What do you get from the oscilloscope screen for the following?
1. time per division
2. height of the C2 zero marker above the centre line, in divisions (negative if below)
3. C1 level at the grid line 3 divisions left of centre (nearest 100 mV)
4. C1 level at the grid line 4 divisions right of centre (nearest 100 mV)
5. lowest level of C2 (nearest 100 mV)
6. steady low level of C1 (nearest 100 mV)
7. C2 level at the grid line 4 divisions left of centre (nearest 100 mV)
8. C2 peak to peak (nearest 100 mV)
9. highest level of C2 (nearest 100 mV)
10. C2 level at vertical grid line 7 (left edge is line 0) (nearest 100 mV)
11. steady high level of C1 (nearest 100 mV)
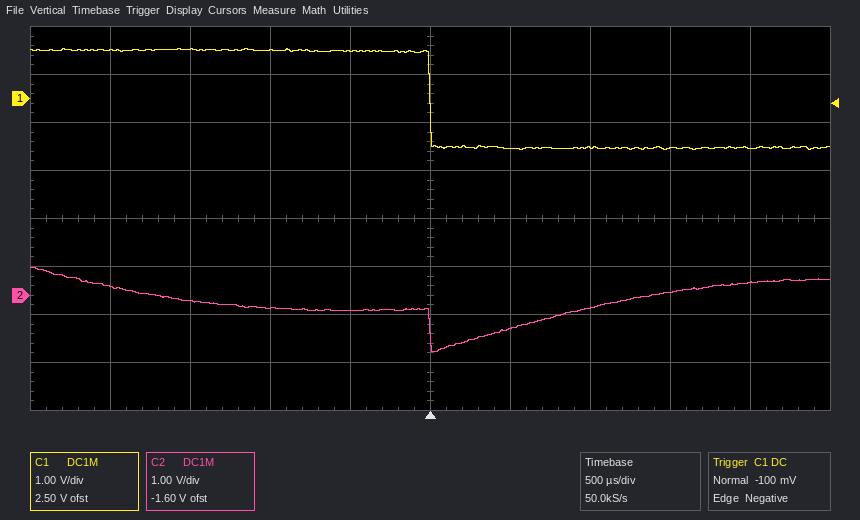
500 µs
-1.6 div
1.0 V
-1.0 V
-1.2 V
-1.0 V
200 mV
1.8 V
600 mV
-300 mV
1.0 V
